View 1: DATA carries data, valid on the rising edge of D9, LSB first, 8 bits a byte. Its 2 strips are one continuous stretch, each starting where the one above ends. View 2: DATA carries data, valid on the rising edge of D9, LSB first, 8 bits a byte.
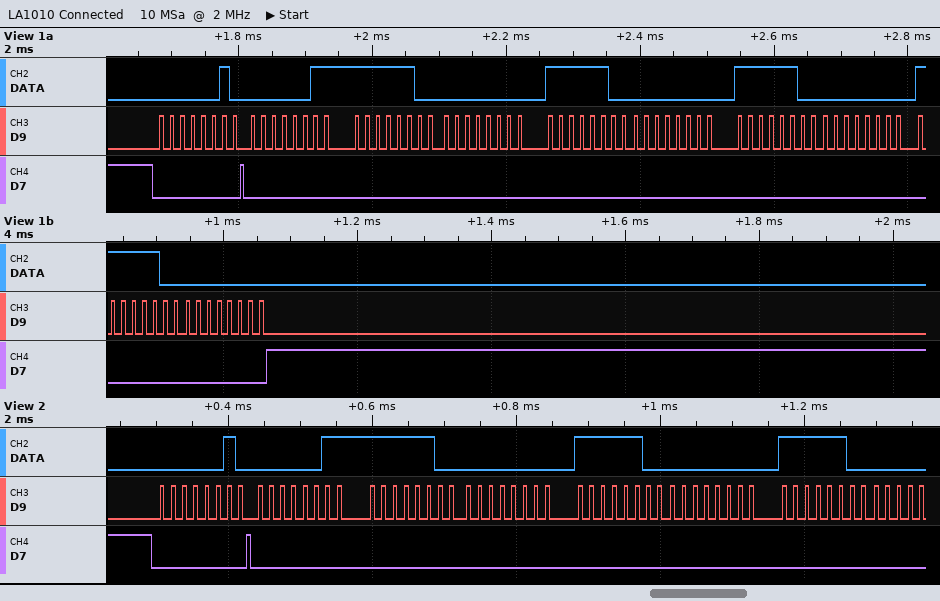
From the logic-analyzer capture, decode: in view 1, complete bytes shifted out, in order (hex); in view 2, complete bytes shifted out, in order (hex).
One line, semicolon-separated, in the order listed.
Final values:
40 C0 3F 00 3F 00 3F 00 3F 00; 0x40 0xC0 0x3F 0x00 0x3F 0x00 0x3F
